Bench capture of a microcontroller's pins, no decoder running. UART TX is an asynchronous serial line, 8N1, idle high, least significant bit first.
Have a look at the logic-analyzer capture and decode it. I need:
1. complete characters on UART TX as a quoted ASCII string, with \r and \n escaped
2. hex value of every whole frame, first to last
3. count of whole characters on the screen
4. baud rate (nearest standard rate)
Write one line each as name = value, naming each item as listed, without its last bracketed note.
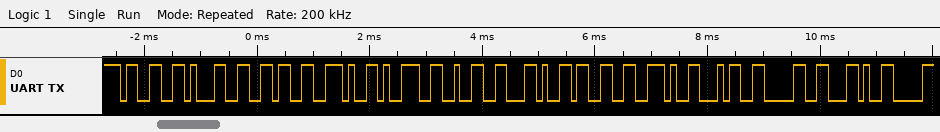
complete characters on UART TX as a quoted ASCII string, with \r and \n escaped = "316.92,3.40,"
hex value of every whole frame, first to last = 0x33 0x31 0x36 0x2E 0x39 0x32 0x2C 0x33 0x2E 0x34 0x30 0x2C
count of whole characters on the screen = 12
baud rate = 9600 baud
